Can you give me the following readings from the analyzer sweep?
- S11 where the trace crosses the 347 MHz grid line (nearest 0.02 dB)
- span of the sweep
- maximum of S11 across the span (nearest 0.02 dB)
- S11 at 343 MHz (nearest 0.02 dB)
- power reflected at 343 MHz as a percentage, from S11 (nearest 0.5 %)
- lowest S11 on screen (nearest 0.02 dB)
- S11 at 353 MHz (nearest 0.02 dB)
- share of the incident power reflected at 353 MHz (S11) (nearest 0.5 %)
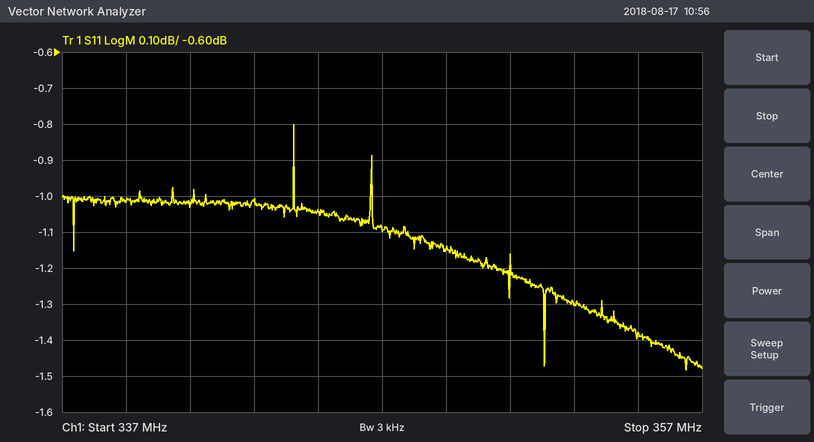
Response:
-1.10 dB
20 MHz
-0.80 dB
-1.02 dB
79.0 %
-1.48 dB
-1.30 dB
74.0 %
